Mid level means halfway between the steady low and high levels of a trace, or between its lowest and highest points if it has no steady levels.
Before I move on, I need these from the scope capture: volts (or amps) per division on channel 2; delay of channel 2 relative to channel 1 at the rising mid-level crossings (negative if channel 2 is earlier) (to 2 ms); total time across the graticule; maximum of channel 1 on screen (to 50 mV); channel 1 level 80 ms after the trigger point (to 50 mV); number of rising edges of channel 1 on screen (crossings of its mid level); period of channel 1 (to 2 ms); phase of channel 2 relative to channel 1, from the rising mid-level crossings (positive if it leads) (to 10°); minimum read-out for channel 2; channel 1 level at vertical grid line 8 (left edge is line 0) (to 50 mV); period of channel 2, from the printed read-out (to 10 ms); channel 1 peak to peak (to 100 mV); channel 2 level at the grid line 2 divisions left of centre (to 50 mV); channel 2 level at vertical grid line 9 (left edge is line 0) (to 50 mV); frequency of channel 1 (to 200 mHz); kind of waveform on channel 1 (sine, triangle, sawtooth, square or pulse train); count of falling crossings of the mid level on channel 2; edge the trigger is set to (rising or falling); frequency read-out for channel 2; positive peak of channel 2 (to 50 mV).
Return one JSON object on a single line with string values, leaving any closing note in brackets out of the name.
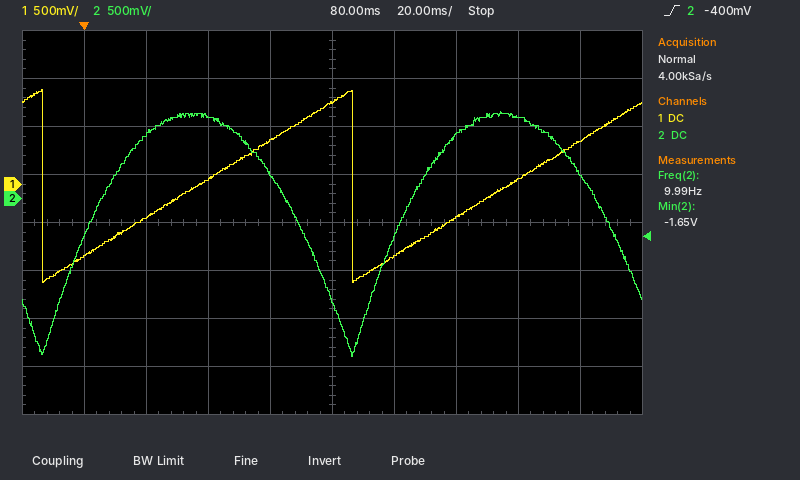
{"volts (or amps) per division on channel 2": "500 mV", "delay of channel 2 relative to channel 1 at the rising mid-level crossings (negative if channel 2 is earlier)": "-36 ms", "total time across the graticule": "200 ms", "maximum of channel 1 on screen": "1.00 V", "channel 1 level 80 ms after the trigger point": "850 mV", "number of rising edges of channel 1 on screen": "2", "period of channel 1": "100 ms", "phase of channel 2 relative to channel 1, from the rising mid-level crossings (positive if it leads)": "+130°", "minimum read-out for channel 2": "-1.65 V", "channel 1 level at vertical grid line 8 (left edge is line 0)": "50 mV", "period of channel 2, from the printed read-out": "100 ms", "channel 1 peak to peak": "2.00 V", "channel 2 level at the grid line 2 divisions left of centre": "850 mV", "channel 2 level at vertical grid line 9 (left edge is line 0)": "250 mV", "frequency of channel 1": "10.0 Hz", "kind of waveform on channel 1": "sawtooth", "count of falling crossings of the mid level on channel 2": "2", "edge the trigger is set to": "rising", "frequency read-out for channel 2": "9.99 Hz", "positive peak of channel 2": "900 mV"}
